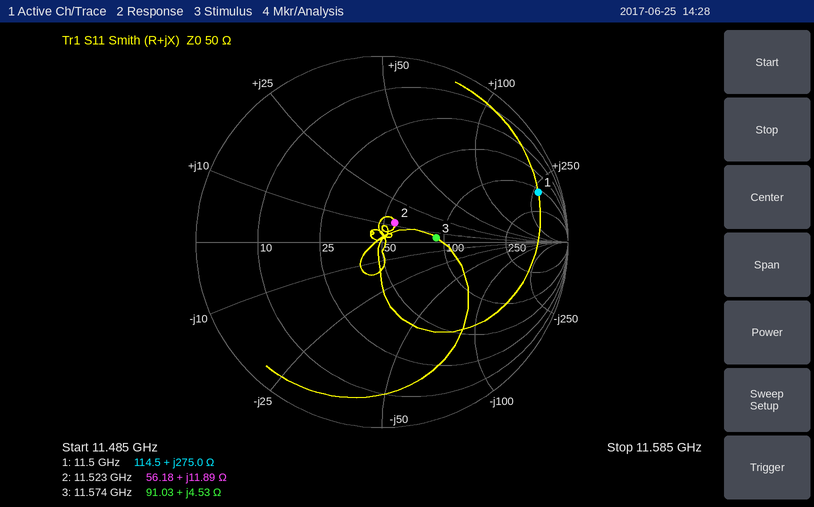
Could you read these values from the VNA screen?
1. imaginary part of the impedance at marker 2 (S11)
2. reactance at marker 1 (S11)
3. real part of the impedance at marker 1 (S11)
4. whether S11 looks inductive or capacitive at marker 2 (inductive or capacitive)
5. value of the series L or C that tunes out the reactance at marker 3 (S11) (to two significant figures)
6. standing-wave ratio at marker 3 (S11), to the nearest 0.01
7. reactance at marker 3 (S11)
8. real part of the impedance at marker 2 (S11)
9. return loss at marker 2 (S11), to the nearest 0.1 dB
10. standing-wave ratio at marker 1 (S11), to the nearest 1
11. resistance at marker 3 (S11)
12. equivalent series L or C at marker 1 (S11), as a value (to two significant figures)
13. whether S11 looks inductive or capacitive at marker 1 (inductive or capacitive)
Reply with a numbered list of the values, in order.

1. +11.89 Ω
2. +275.0 Ω
3. 114.5 Ω
4. inductive
5. 3.0 pF
6. 1.83
7. +4.53 Ω
8. 56.18 Ω
9. 18.0 dB
10. 16
11. 91.03 Ω
12. 3.8 nH
13. inductive
